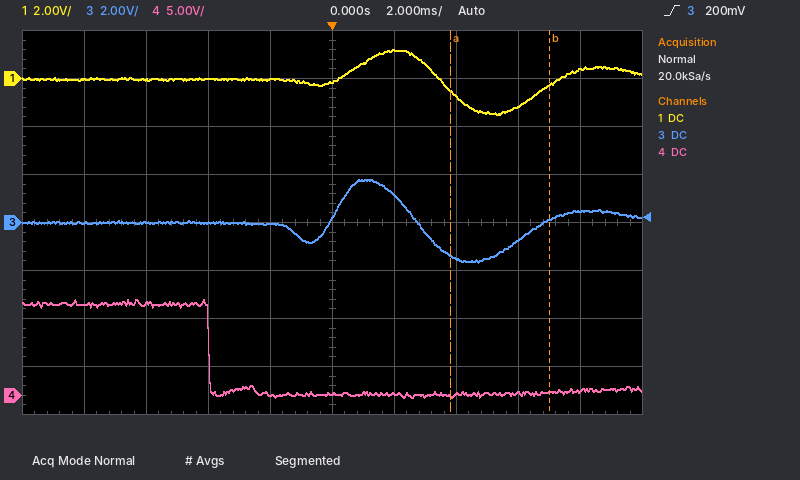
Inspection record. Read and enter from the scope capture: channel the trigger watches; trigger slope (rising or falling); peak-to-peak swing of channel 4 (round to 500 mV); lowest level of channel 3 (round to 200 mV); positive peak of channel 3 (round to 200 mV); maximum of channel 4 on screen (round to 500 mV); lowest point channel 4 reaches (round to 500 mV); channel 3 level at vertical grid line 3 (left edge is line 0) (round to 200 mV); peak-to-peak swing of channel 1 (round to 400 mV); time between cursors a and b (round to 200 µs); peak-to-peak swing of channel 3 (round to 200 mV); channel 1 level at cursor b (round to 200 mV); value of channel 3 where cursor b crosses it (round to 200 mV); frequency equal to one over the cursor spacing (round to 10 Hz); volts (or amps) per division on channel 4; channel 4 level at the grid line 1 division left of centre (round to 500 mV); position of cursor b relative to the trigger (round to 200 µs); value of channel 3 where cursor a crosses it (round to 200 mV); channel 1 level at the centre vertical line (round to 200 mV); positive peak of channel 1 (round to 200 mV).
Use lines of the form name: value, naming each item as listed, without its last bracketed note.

channel the trigger watches: channel 3
trigger slope: rising
peak-to-peak swing of channel 4: 10.0 V
lowest level of channel 3: -1.6 V
positive peak of channel 3: 1.8 V
maximum of channel 4 on screen: 10.0 V
lowest point channel 4 reaches: 0.0 V
channel 3 level at vertical grid line 3 (left edge is line 0): 0.0 V
peak-to-peak swing of channel 1: 2.8 V
time between cursors a and b: 3.2 ms
peak-to-peak swing of channel 3: 3.4 V
channel 1 level at cursor b: -200 mV
value of channel 3 where cursor b crosses it: 200 mV
frequency equal to one over the cursor spacing: 310 Hz
volts (or amps) per division on channel 4: 5 V
channel 4 level at the grid line 1 division left of centre: 0.0 V
position of cursor b relative to the trigger: +7.0 ms
value of channel 3 where cursor a crosses it: -1.4 V
channel 1 level at the centre vertical line: -200 mV
positive peak of channel 1: 1.2 V
